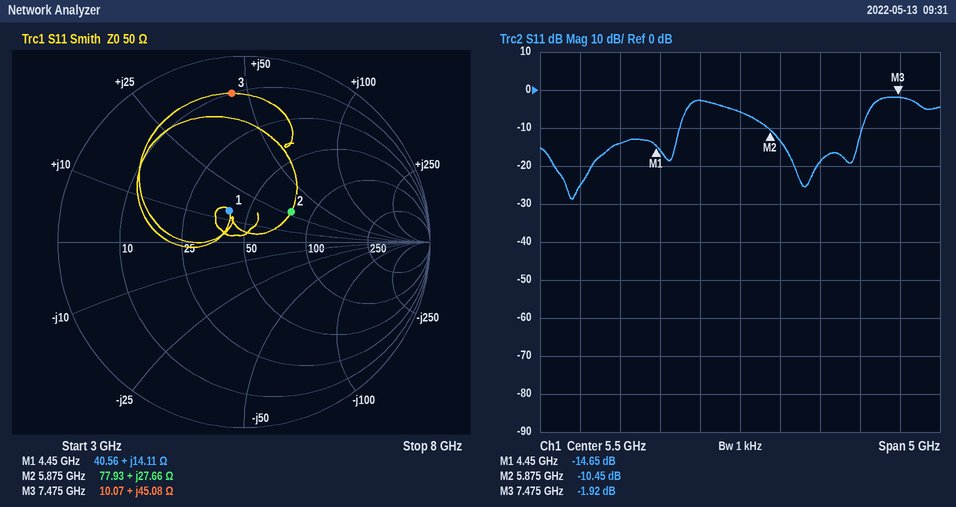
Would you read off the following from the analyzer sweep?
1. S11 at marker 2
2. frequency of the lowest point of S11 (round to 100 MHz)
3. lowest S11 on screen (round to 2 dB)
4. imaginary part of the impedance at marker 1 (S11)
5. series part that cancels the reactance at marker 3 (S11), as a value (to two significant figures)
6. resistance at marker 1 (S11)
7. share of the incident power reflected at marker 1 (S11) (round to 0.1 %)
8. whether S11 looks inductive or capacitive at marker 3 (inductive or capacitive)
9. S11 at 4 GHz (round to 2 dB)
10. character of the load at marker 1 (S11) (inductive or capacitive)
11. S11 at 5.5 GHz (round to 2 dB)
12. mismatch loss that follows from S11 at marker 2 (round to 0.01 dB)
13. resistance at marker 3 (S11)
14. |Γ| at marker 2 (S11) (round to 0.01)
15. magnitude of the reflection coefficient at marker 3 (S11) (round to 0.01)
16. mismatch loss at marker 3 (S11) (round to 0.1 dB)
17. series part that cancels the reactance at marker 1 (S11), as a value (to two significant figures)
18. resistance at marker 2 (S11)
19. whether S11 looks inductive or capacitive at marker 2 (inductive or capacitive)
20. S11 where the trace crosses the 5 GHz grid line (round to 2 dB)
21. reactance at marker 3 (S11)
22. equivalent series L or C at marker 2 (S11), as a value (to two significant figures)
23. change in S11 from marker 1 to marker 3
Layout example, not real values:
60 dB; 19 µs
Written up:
-10.45 dB; 3.4 GHz; -28 dB; +14.11 Ω; 470 fF; 40.56 Ω; 3.4 %; inductive; -14 dB; inductive; -6 dB; 0.41 dB; 10.07 Ω; 0.30; 0.80; 4.5 dB; 2.5 pF; 77.93 Ω; inductive; -2 dB; +45.08 Ω; 750 pH; 12.73 dB
